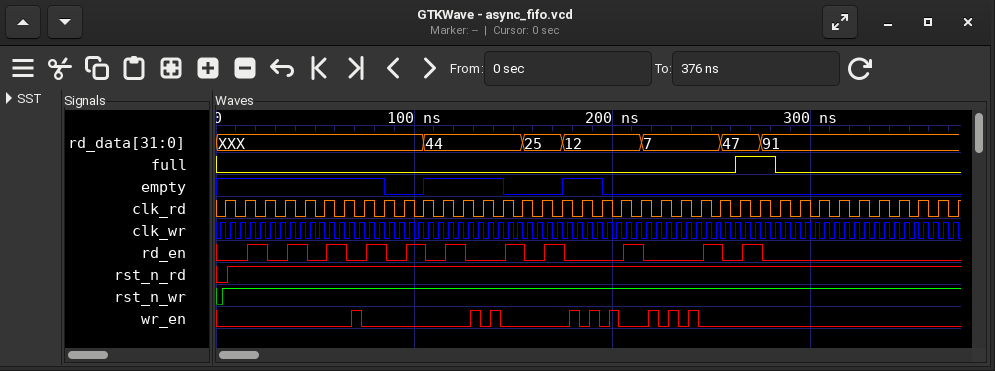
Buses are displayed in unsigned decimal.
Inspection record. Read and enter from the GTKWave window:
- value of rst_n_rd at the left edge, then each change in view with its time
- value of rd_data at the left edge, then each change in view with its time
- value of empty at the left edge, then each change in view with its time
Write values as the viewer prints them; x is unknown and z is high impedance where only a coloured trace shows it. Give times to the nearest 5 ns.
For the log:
0, 1 at 5 ns
XXX, 44 at 105 ns, 25 at 155 ns, 12 at 175 ns, 7 at 215 ns, 47 at 255 ns, 91 at 275 ns
1, 0 at 85 ns, 1 at 105 ns, 0 at 145 ns, 1 at 175 ns, 0 at 195 ns
